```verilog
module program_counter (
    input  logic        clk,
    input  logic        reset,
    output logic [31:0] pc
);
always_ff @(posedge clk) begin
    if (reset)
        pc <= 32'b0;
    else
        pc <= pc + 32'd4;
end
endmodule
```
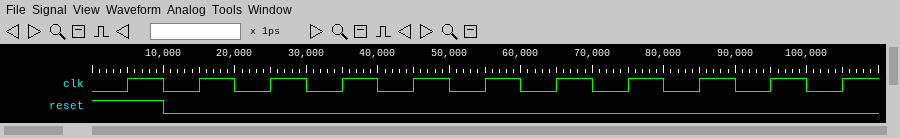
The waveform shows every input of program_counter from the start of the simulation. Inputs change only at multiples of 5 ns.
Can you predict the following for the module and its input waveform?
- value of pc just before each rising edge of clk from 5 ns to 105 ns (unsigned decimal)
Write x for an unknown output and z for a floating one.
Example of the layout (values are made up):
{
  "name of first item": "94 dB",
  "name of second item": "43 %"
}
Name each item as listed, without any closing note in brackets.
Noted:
{
  "value of pc just before each rising edge of clk from 5 ns to 105 ns": "x, 0, 4, 8, 12, 16, 20, 24, 28, 32, 36"
}
